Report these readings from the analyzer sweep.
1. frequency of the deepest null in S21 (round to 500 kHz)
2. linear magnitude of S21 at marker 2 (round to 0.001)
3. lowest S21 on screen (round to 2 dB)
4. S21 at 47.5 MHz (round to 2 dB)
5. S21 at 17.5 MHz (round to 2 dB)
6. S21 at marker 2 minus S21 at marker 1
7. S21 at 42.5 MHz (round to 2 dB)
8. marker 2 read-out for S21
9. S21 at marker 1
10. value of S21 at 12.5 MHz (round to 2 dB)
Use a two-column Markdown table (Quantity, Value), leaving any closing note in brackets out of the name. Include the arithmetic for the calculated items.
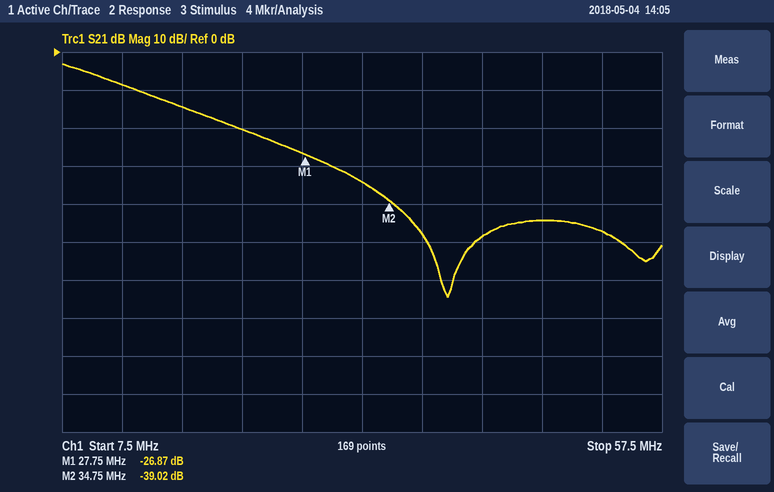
| Quantity | Value |
|---|---|
| frequency of the deepest null in S21 | 39.5 MHz |
| linear magnitude of S21 at marker 2 | 10^(-39.02/20) ≈ 0.011 |
| lowest S21 on screen | -64 dB |
| S21 at 47.5 MHz | -44 dB |
| S21 at 17.5 MHz | -14 dB |
| S21 at marker 2 minus S21 at marker 1 | -39.02 − (-26.87) = -12.15 dB |
| S21 at 42.5 MHz | -48 dB |
| marker 2 read-out for S21 | -39.02 dB |
| S21 at marker 1 | -26.87 dB |
| value of S21 at 12.5 MHz | -8 dB |
